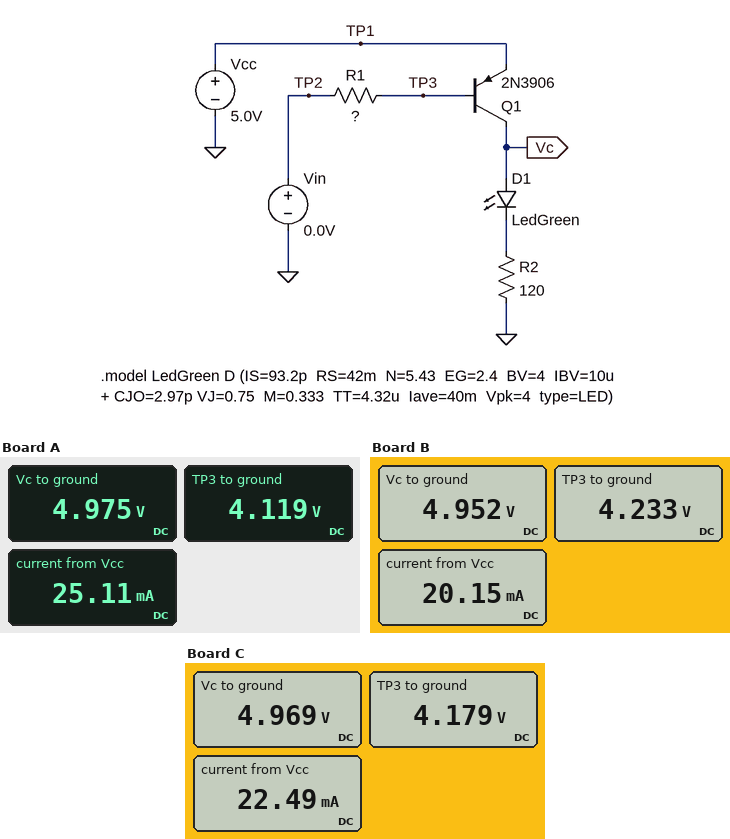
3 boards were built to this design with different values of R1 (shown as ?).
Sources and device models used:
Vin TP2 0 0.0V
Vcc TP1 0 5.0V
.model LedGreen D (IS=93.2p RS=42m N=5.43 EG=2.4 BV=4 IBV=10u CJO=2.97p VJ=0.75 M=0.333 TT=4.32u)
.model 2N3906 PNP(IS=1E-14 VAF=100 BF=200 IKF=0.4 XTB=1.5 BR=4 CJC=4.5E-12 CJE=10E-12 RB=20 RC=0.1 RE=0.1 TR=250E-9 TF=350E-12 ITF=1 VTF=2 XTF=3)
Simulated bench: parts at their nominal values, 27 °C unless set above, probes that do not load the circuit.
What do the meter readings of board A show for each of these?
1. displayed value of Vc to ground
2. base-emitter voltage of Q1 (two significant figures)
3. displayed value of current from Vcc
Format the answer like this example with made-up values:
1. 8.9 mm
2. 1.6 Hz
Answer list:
1. 4.975 V
2. -880 mV
3. 25.11 mA
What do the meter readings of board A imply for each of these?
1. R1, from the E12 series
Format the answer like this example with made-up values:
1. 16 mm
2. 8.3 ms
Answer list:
1. 680 Ω
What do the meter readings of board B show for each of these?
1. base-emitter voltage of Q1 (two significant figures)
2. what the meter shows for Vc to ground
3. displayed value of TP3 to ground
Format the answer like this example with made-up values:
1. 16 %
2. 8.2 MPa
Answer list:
1. -770 mV
2. 4.952 V
3. 4.233 V
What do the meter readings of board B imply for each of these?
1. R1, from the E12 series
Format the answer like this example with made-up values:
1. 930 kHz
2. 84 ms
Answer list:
1. 3.3 kΩ
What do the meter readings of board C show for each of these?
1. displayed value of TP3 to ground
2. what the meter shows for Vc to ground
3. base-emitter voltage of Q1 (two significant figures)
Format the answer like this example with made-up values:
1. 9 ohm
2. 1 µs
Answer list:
1. 4.179 V
2. 4.969 V
3. -820 mV
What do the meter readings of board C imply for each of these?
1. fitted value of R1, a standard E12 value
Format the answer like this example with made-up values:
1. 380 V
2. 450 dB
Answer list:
1. 1.2 kΩ
